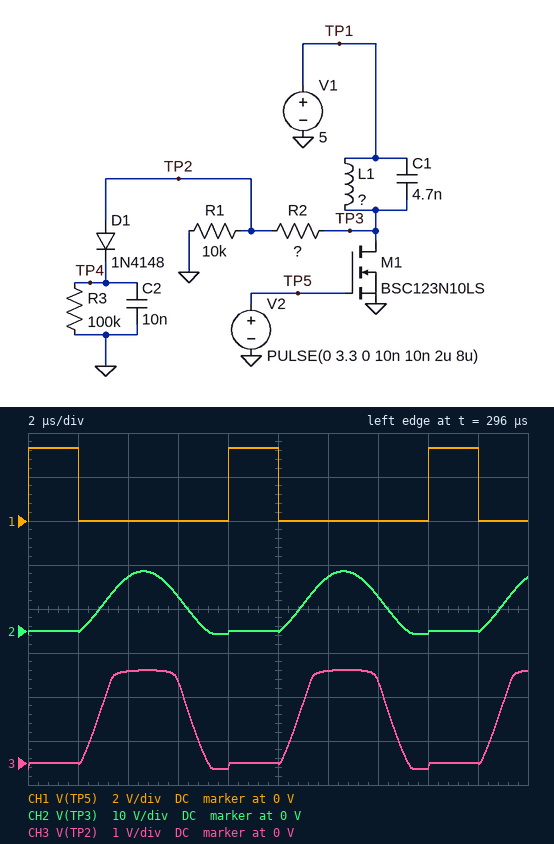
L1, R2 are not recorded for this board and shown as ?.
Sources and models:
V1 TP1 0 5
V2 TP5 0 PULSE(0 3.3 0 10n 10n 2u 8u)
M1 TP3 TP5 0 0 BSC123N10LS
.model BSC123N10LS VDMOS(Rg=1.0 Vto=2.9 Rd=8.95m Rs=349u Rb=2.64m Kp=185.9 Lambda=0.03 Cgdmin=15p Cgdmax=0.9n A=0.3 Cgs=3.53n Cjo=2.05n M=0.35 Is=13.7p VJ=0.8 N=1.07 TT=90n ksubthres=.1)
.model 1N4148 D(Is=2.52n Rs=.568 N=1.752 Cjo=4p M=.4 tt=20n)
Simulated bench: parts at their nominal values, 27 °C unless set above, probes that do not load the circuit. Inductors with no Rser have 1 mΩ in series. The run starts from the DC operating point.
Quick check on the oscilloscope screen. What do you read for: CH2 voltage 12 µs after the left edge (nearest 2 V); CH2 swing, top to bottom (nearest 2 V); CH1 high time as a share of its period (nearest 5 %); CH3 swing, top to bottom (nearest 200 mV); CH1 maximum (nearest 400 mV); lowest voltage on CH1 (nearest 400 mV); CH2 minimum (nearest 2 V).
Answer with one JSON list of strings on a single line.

["12 V", "14 V", "25 %", "2.2 V", "3.2 V", "0 V", "0 V"]
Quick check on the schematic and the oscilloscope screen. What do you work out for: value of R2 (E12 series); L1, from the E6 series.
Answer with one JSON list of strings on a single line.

["33 kΩ", "220 µH"]
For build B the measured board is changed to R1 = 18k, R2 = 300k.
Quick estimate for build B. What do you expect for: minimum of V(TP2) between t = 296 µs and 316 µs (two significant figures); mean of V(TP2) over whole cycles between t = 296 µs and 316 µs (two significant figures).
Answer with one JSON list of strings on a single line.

["-33 mV", "230 mV"]
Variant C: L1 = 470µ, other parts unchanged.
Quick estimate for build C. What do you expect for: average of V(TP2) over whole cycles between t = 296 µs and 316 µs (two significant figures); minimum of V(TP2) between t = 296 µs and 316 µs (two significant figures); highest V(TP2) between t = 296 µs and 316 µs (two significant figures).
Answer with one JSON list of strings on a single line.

["990 mV", "-50 mV", "1.9 V"]
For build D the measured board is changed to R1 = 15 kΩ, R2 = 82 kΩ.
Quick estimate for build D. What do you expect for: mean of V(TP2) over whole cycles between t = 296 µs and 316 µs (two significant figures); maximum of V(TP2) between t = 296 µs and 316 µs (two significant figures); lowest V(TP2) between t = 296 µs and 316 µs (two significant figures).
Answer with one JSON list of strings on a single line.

["580 mV", "1.3 V", "-91 mV"]
